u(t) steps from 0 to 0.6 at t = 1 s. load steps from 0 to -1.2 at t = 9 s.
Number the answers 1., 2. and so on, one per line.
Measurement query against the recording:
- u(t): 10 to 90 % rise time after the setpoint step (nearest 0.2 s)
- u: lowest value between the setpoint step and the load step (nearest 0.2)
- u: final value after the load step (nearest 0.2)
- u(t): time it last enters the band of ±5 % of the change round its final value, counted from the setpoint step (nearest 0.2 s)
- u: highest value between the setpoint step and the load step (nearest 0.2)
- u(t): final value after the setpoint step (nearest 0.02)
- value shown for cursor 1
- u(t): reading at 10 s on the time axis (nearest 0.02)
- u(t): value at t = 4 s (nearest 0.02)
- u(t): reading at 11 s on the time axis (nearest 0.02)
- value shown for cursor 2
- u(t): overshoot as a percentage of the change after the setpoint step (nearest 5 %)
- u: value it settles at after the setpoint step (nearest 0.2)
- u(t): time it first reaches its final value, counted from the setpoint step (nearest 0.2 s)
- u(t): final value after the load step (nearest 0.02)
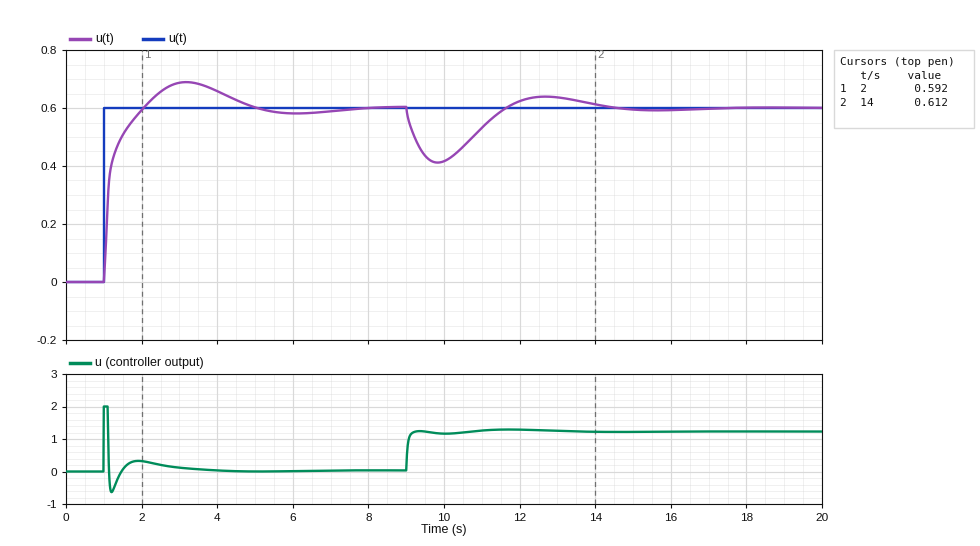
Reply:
1. 0.6 s
2. -0.6
3. 1.2
4. 3.4 s
5. 2.0
6. 0.60
7. 0.592
8. 0.42
9. 0.66
10. 0.54
11. 0.612
12. 15 %
13. 0.0
14. 1.0 s
15. 0.60
